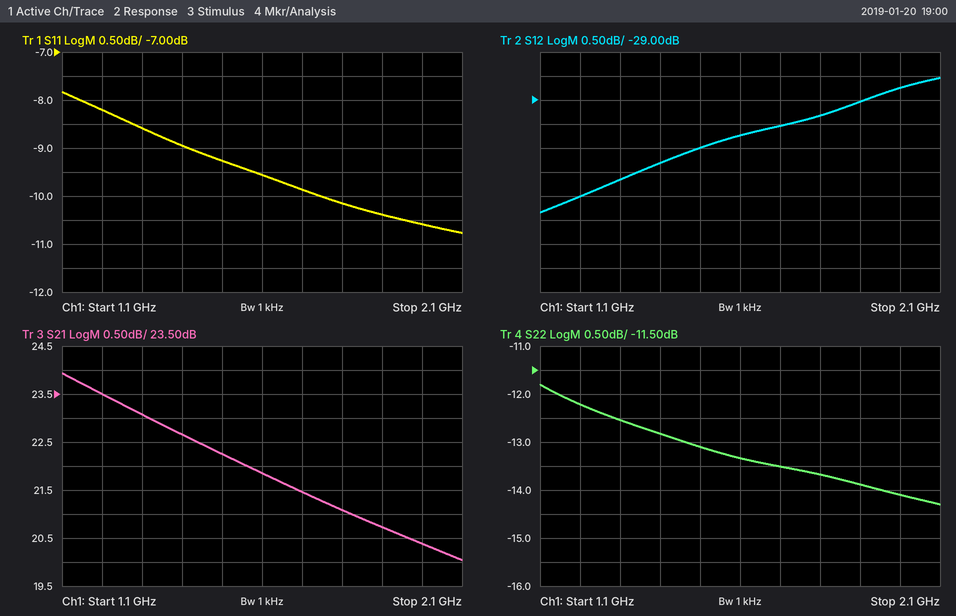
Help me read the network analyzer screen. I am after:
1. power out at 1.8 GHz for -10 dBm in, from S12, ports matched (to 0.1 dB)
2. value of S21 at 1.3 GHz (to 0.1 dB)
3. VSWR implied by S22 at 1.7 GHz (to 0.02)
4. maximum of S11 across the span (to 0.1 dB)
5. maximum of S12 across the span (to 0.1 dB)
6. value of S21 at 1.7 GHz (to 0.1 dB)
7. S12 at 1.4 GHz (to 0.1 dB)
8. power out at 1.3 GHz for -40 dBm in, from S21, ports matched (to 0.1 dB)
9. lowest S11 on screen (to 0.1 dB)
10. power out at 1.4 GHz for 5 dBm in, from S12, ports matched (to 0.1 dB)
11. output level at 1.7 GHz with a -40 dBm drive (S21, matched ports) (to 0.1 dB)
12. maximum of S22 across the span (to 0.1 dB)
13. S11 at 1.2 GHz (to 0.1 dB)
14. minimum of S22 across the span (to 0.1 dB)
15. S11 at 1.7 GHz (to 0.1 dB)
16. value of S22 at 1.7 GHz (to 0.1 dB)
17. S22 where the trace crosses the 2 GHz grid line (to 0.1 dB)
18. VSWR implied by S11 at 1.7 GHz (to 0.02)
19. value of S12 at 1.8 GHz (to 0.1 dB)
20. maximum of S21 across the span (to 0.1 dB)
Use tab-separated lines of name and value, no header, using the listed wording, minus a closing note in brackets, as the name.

power out at 1.8 GHz for -10 dBm in, from S12, ports matched	-39.3 dBm
value of S21 at 1.3 GHz	23.1 dB
VSWR implied by S22 at 1.7 GHz	1.54
maximum of S11 across the span	-7.8 dB
maximum of S12 across the span	-28.5 dB
value of S21 at 1.7 GHz	21.5 dB
S12 at 1.4 GHz	-30.3 dB
power out at 1.3 GHz for -40 dBm in, from S21, ports matched	-16.9 dBm
lowest S11 on screen	-10.8 dB
power out at 1.4 GHz for 5 dBm in, from S12, ports matched	-25.3 dBm
output level at 1.7 GHz with a -40 dBm drive (S21, matched ports)	-18.5 dBm
maximum of S22 across the span	-11.8 dB
S11 at 1.2 GHz	-8.2 dB
minimum of S22 across the span	-14.3 dB
S11 at 1.7 GHz	-9.9 dB
value of S22 at 1.7 GHz	-13.5 dB
S22 where the trace crosses the 2 GHz grid line	-14.1 dB
VSWR implied by S11 at 1.7 GHz	1.94
value of S12 at 1.8 GHz	-29.3 dB
maximum of S21 across the span	23.9 dB
